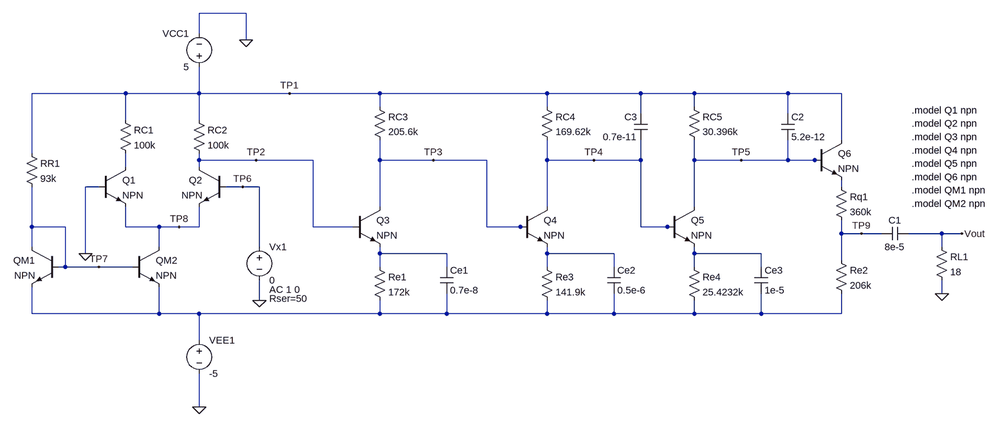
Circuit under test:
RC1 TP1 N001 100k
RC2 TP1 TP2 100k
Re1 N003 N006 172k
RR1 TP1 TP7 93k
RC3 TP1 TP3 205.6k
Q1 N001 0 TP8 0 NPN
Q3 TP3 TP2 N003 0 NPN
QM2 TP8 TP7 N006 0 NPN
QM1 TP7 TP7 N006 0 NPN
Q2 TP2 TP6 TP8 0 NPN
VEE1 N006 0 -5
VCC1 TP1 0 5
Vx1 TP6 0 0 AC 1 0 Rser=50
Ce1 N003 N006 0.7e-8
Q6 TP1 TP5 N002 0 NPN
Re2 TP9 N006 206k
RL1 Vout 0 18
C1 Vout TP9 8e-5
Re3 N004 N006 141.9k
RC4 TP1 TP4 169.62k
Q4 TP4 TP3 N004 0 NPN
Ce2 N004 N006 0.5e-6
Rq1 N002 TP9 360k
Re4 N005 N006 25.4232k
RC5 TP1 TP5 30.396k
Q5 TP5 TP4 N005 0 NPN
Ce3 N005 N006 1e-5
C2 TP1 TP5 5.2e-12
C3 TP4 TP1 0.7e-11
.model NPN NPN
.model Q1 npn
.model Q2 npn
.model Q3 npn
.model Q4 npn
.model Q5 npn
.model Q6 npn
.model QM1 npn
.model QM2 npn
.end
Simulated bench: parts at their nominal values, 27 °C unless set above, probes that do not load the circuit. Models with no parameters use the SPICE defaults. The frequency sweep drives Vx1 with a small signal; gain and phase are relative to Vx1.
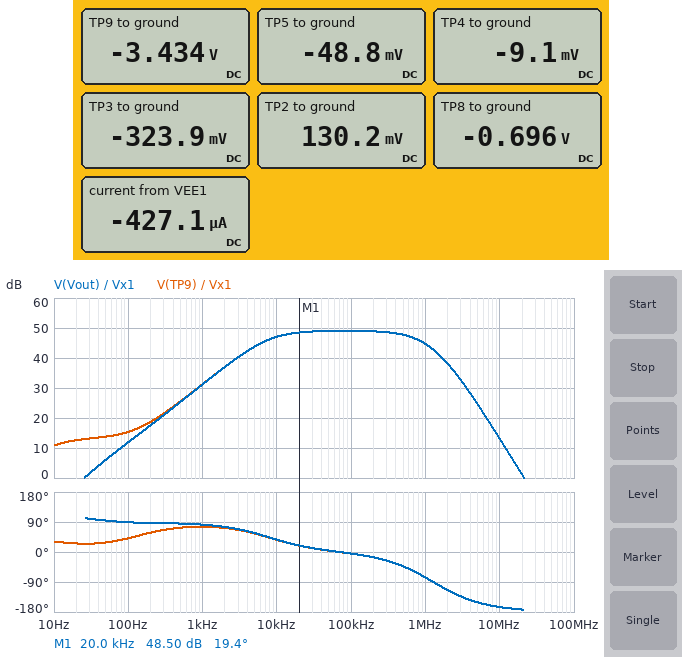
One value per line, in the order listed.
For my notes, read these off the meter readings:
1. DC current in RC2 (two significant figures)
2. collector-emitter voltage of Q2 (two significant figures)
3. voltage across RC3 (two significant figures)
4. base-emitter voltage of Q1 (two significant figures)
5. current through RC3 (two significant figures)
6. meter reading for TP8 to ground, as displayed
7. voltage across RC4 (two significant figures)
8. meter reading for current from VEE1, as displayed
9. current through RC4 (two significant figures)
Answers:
49 µA
830 mV
5.3 V
700 mV
26 µA
-0.696 V
5.0 V
-427.1 µA
30 µA
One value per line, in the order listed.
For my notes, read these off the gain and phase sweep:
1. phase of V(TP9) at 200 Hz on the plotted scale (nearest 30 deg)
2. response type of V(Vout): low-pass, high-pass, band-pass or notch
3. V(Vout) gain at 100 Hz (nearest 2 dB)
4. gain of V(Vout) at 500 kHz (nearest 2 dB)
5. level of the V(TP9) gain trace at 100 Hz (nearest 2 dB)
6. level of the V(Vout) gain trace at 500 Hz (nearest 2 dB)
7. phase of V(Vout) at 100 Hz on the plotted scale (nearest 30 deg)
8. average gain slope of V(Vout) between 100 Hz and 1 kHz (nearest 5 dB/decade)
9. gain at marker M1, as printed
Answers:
60 deg
band-pass
12 dB
48 dB
16 dB
26 dB
90 deg
20 dB/decade
48.50 dB
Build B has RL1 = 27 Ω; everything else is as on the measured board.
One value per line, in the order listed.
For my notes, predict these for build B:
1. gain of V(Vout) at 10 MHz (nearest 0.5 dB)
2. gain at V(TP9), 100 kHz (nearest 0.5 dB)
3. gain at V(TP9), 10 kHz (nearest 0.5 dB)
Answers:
16.5 dB
52.5 dB
50.5 dB
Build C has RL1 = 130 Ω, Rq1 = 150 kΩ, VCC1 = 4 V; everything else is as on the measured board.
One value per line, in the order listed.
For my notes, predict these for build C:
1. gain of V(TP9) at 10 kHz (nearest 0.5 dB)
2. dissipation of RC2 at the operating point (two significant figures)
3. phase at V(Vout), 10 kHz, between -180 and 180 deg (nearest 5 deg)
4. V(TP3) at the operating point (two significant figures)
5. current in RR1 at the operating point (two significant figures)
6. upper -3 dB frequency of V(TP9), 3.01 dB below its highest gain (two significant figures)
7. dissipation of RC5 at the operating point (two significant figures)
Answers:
72.0 dB
190 µW
45 deg
-760 mV
89 µA
770 kHz
670 µW
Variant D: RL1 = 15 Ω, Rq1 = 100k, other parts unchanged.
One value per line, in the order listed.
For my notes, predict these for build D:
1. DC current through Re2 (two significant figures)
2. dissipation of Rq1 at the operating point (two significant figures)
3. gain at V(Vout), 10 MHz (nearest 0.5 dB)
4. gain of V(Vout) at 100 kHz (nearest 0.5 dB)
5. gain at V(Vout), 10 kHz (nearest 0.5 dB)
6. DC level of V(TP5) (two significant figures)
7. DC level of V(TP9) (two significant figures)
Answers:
14 µA
20 µW
22.5 dB
58.5 dB
56.5 dB
-51 mV
-2.1 V
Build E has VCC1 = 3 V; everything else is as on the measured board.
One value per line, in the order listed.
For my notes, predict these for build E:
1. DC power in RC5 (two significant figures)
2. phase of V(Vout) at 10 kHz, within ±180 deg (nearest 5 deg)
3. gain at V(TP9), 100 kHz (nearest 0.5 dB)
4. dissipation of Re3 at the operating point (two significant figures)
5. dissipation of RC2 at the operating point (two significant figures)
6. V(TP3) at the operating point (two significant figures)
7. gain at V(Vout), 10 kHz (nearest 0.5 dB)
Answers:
530 µW
25 deg
-3.0 dB
68 µW
130 µW
-1.2 V
-3.5 dB
